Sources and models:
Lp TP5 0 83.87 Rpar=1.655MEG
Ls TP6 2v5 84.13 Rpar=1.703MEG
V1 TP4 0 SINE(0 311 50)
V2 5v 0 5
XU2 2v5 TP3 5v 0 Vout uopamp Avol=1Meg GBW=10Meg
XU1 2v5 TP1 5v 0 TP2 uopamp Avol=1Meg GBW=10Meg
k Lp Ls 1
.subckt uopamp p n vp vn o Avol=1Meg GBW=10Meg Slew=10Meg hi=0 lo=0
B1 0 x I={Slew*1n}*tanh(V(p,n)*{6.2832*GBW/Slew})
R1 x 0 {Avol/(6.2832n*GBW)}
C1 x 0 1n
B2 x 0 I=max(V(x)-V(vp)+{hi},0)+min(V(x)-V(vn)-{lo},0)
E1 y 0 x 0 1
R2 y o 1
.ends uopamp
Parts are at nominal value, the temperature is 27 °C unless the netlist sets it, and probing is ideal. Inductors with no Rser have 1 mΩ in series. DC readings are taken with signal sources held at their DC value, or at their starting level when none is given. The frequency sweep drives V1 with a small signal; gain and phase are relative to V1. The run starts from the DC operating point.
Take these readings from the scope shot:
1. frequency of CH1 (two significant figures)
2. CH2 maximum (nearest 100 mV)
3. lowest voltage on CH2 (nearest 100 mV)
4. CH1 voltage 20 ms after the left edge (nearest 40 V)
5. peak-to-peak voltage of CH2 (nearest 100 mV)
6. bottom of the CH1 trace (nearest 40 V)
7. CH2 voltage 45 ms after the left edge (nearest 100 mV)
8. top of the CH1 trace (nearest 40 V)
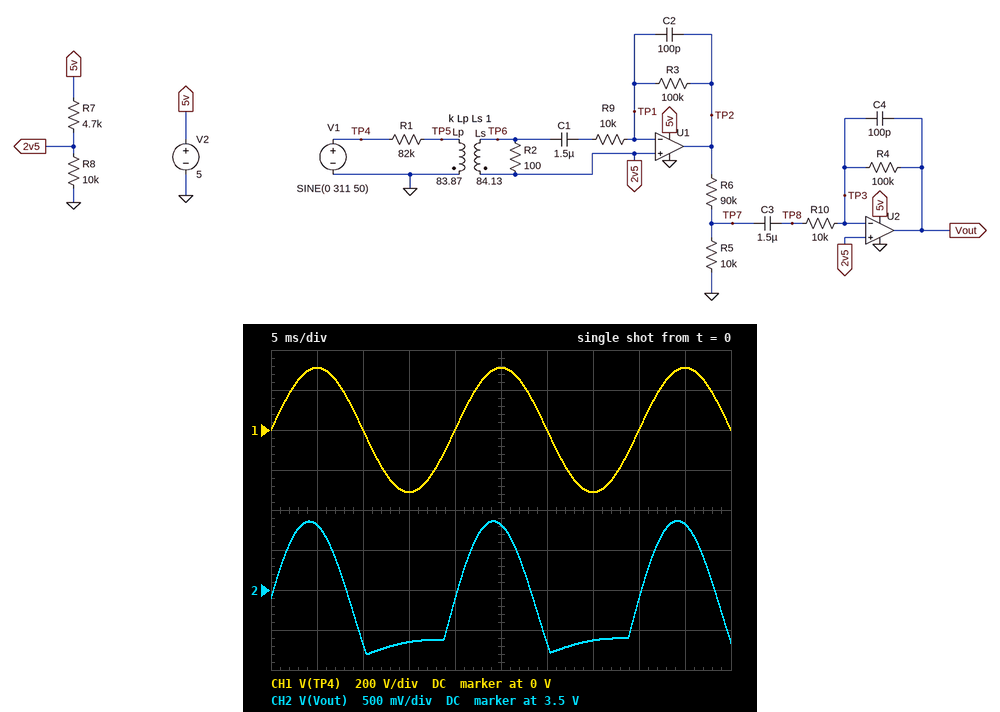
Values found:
50 Hz
4.4 V
2.7 V
0 V
1.7 V
-320 V
4.3 V
320 V
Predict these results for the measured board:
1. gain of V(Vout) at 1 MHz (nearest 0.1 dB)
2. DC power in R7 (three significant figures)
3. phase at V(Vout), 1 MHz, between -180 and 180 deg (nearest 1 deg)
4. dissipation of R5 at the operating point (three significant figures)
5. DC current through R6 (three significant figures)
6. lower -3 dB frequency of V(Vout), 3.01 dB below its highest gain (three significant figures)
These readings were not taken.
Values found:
-68.5 dB
544 µW
168 deg
11.6 µW
34.0 µA
12.7 Hz
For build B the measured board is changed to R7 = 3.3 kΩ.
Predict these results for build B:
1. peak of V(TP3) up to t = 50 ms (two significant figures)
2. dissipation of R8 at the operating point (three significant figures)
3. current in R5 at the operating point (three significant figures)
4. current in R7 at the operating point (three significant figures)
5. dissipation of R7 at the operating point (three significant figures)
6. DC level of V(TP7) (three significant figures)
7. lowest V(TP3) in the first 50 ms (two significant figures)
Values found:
3.8 V
1.41 mW
37.6 µA
376 µA
466 µW
376 mV
3.7 V
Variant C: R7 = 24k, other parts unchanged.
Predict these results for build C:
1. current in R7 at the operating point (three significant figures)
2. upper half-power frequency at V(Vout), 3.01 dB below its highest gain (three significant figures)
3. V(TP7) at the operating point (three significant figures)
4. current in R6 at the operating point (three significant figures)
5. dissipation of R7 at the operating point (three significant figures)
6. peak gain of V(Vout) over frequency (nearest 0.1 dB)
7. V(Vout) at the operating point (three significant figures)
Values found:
147 µA
39.2 kHz
147 mV
14.7 µA
519 µW
-50.3 dB
1.47 V
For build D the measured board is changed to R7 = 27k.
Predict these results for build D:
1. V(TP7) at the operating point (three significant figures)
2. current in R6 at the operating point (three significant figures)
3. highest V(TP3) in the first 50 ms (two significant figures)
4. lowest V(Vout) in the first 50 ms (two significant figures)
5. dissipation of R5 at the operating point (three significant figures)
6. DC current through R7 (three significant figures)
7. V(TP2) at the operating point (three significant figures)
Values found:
135 mV
13.5 µA
1.6 V
990 mV
1.83 µW
135 µA
1.35 V
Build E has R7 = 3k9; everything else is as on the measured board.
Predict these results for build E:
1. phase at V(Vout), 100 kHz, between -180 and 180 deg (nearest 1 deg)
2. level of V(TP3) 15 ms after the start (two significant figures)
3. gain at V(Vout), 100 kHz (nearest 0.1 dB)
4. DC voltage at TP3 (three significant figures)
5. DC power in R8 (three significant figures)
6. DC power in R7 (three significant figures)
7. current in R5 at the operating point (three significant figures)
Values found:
158 deg
3.6 V
-65.2 dB
3.60 V
1.29 mW
505 µW
36.0 µA
